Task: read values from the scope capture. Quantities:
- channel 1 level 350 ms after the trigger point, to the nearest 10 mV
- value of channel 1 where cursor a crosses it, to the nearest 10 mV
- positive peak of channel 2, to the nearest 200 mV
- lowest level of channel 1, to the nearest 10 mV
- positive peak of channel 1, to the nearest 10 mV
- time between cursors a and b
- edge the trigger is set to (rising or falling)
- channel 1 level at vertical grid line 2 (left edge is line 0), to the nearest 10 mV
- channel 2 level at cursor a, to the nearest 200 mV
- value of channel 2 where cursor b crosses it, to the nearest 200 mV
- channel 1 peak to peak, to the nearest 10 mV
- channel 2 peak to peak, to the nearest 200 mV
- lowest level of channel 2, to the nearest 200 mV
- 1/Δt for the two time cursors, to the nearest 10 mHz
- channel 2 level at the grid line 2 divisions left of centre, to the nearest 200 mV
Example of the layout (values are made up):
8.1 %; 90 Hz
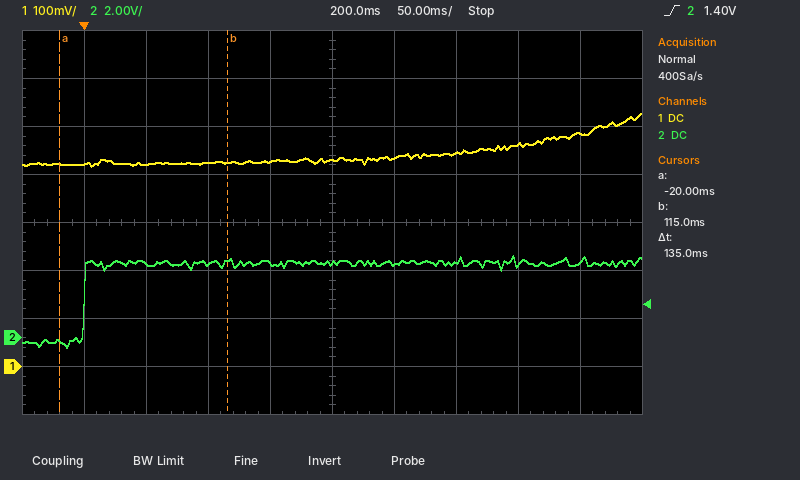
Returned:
460 mV; 420 mV; 3.4 V; 420 mV; 530 mV; 135 ms; rising; 420 mV; -200 mV; 3.2 V; 110 mV; 3.8 V; -400 mV; 7.41 Hz; 3.0 V
